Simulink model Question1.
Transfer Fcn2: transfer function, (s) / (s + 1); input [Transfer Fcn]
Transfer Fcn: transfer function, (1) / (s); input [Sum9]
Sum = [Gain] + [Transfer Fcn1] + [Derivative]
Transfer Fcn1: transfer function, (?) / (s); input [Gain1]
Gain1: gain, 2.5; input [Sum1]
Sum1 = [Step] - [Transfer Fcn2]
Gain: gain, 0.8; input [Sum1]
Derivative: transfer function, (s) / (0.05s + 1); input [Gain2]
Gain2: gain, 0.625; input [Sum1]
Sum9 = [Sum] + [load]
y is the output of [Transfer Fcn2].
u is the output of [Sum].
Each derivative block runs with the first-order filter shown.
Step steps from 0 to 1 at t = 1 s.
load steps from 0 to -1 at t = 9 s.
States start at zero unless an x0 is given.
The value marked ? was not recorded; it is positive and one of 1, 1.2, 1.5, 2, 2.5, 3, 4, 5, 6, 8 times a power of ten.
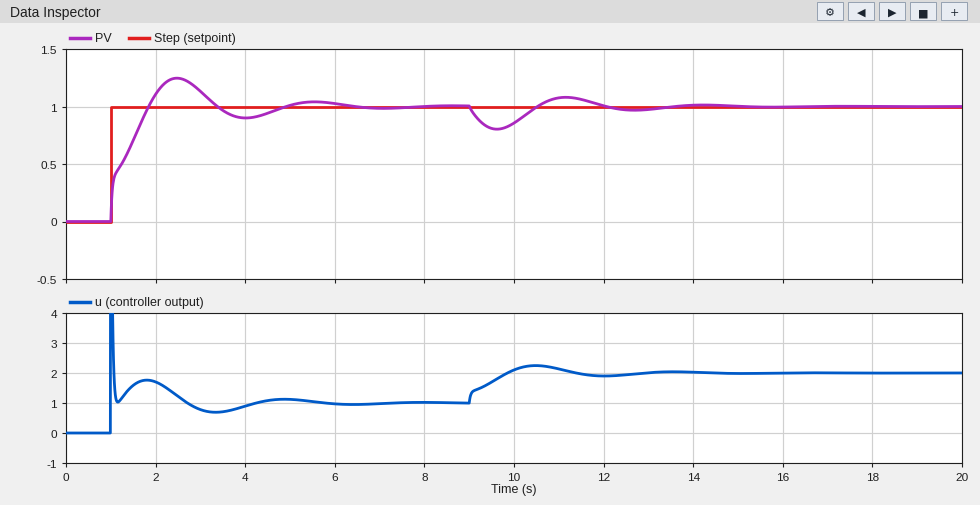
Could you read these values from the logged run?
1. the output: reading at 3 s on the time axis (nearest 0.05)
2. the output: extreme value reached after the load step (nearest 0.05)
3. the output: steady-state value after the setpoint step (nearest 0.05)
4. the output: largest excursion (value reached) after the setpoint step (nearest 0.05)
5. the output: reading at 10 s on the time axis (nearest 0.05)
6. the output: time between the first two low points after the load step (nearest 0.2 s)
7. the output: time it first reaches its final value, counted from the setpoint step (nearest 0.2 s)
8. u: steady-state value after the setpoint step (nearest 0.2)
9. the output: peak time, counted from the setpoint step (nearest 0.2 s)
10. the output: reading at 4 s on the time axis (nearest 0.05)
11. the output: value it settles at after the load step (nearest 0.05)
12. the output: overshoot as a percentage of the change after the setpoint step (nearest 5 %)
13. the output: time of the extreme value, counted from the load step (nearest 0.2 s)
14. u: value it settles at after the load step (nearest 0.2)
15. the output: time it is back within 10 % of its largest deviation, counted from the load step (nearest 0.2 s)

1.15
0.80
1.00
1.25
0.85
3.0 s
0.8 s
1.0
1.4 s
0.90
1.00
25 %
0.6 s
2.0
4.2 s
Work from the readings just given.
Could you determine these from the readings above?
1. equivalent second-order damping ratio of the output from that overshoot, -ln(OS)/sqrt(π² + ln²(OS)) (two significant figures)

0.40
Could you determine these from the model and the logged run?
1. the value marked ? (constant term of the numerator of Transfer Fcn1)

3
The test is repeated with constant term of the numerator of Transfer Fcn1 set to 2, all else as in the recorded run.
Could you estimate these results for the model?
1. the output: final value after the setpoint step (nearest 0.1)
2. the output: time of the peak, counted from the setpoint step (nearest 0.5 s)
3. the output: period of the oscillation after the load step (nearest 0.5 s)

1.0
2.0 s
4.0 s
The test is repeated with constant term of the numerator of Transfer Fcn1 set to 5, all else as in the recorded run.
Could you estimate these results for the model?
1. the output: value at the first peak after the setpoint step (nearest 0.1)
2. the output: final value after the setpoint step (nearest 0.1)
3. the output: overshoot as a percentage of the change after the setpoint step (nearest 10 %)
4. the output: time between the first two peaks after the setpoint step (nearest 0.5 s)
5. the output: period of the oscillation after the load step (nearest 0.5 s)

1.3
1.0
30 %
2.5 s
2.5 s
